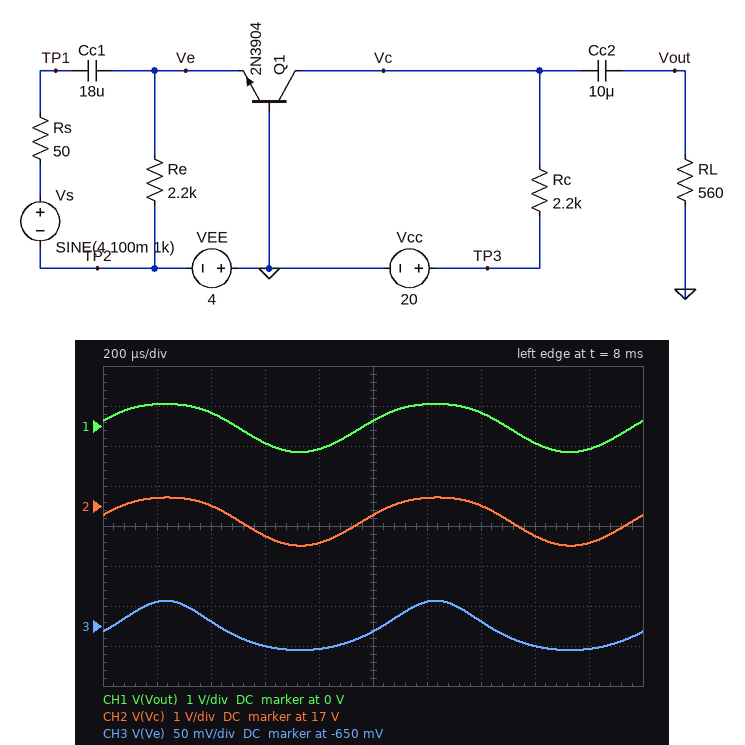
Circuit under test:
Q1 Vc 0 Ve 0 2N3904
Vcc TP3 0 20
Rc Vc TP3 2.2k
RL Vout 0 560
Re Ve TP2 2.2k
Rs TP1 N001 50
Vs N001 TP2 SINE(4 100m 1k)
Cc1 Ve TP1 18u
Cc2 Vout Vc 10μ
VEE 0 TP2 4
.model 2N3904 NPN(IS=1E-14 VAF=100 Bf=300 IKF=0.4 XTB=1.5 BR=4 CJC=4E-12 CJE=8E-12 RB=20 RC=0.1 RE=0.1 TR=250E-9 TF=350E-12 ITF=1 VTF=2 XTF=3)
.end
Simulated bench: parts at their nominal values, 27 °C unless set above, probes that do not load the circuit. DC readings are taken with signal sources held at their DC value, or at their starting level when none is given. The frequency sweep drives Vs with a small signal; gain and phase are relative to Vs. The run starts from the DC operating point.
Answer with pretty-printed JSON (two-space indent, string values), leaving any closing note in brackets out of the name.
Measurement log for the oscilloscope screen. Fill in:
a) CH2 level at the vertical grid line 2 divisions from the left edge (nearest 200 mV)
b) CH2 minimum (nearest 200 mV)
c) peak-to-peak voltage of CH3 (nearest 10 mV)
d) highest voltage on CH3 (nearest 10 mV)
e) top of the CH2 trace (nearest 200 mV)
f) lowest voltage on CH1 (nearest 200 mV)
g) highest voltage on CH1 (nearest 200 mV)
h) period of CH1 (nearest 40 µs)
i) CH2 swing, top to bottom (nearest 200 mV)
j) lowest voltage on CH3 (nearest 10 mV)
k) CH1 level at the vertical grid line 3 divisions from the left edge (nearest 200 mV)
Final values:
{
  "CH2 level at the vertical grid line 2 divisions from the left edge": "17.0 V",
  "CH2 minimum": "16.0 V",
  "peak-to-peak voltage of CH3": "60 mV",
  "highest voltage on CH3": "-620 mV",
  "top of the CH2 trace": "17.2 V",
  "lowest voltage on CH1": "-600 mV",
  "highest voltage on CH1": "600 mV",
  "period of CH1": "1.00 ms",
  "CH2 swing, top to bottom": "1.2 V",
  "lowest voltage on CH3": "-680 mV",
  "CH1 level at the vertical grid line 3 divisions from the left edge": "-400 mV"
}
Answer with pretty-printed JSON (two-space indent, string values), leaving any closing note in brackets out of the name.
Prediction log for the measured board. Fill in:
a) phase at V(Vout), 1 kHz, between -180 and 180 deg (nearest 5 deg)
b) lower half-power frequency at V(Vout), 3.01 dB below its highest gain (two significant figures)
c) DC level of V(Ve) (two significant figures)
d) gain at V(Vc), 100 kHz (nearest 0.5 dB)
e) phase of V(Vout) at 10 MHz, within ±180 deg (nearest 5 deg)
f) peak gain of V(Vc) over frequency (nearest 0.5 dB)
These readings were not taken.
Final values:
{
  "phase at V(Vout), 1 kHz, between -180 and 180 deg": "10 deg",
  "lower half-power frequency at V(Vout), 3.01 dB below its highest gain": "130 Hz",
  "DC level of V(Ve)": "-660 mV",
  "gain at V(Vc), 100 kHz": "16.5 dB",
  "phase of V(Vout) at 10 MHz, within ±180 deg": "-5 deg",
  "peak gain of V(Vc) over frequency": "16.5 dB"
}
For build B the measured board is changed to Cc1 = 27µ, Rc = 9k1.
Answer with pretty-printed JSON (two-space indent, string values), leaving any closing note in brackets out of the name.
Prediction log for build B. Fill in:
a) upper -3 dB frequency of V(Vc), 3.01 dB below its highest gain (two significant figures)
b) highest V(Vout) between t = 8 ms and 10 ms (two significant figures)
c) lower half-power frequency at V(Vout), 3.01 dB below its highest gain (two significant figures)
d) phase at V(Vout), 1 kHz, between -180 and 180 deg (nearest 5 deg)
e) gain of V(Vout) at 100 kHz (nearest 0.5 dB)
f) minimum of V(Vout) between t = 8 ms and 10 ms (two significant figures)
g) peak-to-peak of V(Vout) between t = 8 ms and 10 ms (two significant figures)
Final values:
{
  "upper -3 dB frequency of V(Vc), 3.01 dB below its highest gain": "96 MHz",
  "highest V(Vout) between t = 8 ms and 10 ms": "650 mV",
  "lower half-power frequency at V(Vout), 3.01 dB below its highest gain": "88 Hz",
  "phase at V(Vout), 1 kHz, between -180 and 180 deg": "5 deg",
  "gain of V(Vout) at 100 kHz": "18.0 dB",
  "minimum of V(Vout) between t = 8 ms and 10 ms": "-780 mV",
  "peak-to-peak of V(Vout) between t = 8 ms and 10 ms": "1.4 V"
}
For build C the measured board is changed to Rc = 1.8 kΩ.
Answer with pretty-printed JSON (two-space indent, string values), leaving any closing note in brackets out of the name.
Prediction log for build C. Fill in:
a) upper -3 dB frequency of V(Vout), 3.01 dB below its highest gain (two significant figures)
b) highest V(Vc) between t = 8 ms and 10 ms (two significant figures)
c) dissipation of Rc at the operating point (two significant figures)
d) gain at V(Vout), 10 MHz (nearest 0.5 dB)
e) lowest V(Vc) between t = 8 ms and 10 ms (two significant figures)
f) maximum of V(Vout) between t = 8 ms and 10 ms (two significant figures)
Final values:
{
  "upper -3 dB frequency of V(Vout), 3.01 dB below its highest gain": "140 MHz",
  "highest V(Vc) between t = 8 ms and 10 ms": "18 V",
  "dissipation of Rc at the operating point": "4.1 mW",
  "gain at V(Vout), 10 MHz": "16.0 dB",
  "lowest V(Vc) between t = 8 ms and 10 ms": "17 V",
  "maximum of V(Vout) between t = 8 ms and 10 ms": "530 mV"
}
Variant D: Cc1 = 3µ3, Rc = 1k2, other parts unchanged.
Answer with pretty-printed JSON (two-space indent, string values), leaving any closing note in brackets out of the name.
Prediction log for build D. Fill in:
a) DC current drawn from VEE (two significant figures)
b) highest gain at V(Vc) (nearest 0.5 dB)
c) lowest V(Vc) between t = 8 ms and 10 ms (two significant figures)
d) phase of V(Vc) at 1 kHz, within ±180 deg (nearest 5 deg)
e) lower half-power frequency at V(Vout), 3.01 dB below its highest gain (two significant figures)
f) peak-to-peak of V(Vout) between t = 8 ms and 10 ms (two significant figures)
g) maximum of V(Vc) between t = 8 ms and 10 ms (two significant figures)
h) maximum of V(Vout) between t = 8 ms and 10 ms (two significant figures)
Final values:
{
  "DC current drawn from VEE": "1.5 mA",
  "highest gain at V(Vc)": "15.0 dB",
  "lowest V(Vc) between t = 8 ms and 10 ms": "18 V",
  "phase of V(Vc) at 1 kHz, within ±180 deg": "35 deg",
  "lower half-power frequency at V(Vout), 3.01 dB below its highest gain": "720 Hz",
  "peak-to-peak of V(Vout) between t = 8 ms and 10 ms": "880 mV",
  "maximum of V(Vc) between t = 8 ms and 10 ms": "19 V",
  "maximum of V(Vout) between t = 8 ms and 10 ms": "410 mV"
}
